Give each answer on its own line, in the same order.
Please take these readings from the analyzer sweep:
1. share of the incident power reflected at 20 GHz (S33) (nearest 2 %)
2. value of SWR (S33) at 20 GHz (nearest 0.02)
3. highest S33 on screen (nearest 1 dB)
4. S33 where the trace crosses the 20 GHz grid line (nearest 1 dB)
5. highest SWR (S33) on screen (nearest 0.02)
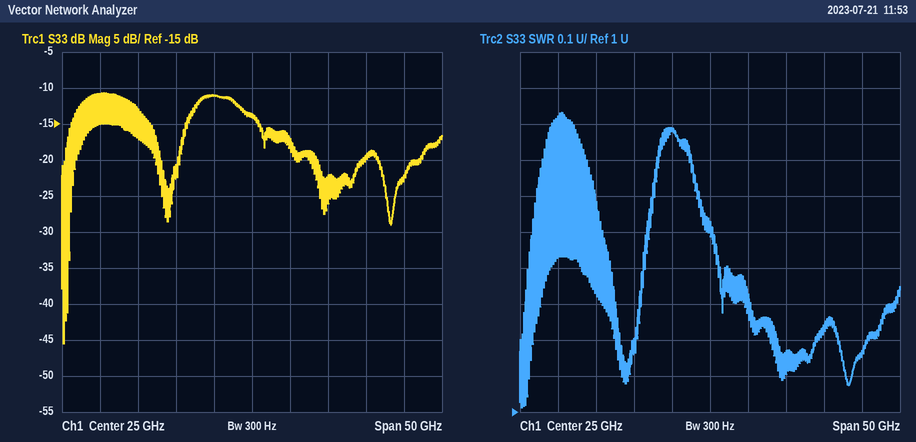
8 %
1.78
-11 dB
-11 dB
1.84
